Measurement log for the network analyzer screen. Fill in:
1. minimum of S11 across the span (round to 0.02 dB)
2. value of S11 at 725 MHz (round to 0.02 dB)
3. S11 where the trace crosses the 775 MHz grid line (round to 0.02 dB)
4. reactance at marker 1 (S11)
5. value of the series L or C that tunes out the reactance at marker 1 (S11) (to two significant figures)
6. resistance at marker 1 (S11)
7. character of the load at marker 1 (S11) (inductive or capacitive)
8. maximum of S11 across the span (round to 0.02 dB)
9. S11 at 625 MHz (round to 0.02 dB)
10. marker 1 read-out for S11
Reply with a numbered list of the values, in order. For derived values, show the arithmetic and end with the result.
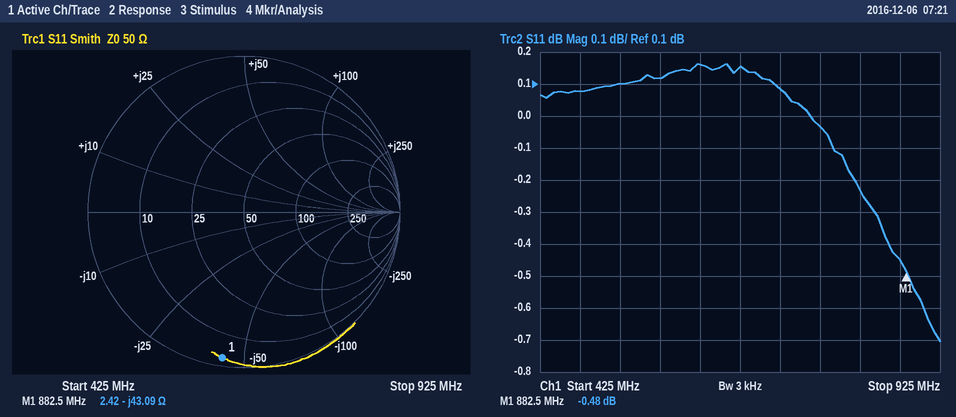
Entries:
1. -0.70 dB
2. 0.08 dB
3. -0.04 dB
4. -43.09 Ω
5. L = 43.09 Ω/(2π × 882.5 MHz) ≈ 7.8 nH
6. 2.42 Ω
7. capacitive
8. 0.16 dB
9. 0.16 dB
10. -0.48 dB
